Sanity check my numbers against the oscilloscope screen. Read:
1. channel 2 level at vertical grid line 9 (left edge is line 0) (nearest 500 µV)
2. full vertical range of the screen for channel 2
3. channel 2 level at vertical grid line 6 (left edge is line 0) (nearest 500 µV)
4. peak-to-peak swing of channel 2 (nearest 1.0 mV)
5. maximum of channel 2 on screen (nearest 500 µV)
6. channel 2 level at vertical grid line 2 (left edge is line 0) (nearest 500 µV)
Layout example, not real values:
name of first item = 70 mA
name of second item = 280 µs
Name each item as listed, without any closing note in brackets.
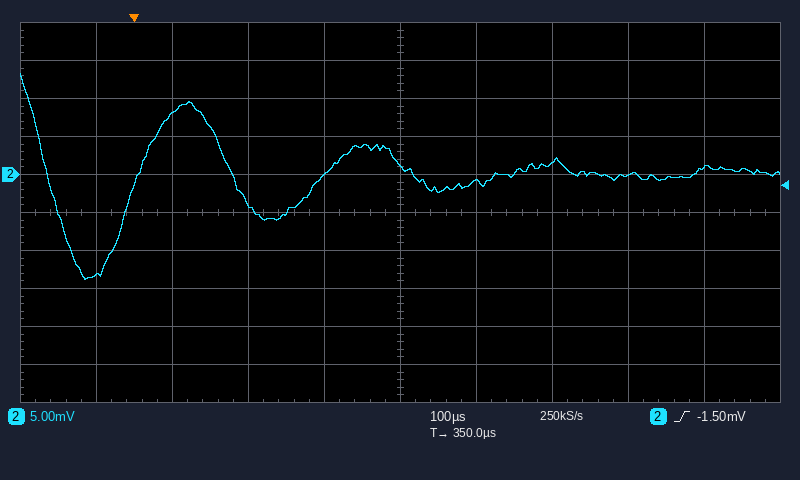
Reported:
channel 2 level at vertical grid line 9 (left edge is line 0) = 1.0 mV
full vertical range of the screen for channel 2 = 50 mV
channel 2 level at vertical grid line 6 (left edge is line 0) = -1.0 mV
peak-to-peak swing of channel 2 = 27.0 mV
maximum of channel 2 on screen = 13.5 mV
channel 2 level at vertical grid line 2 (left edge is line 0) = 8.0 mV
